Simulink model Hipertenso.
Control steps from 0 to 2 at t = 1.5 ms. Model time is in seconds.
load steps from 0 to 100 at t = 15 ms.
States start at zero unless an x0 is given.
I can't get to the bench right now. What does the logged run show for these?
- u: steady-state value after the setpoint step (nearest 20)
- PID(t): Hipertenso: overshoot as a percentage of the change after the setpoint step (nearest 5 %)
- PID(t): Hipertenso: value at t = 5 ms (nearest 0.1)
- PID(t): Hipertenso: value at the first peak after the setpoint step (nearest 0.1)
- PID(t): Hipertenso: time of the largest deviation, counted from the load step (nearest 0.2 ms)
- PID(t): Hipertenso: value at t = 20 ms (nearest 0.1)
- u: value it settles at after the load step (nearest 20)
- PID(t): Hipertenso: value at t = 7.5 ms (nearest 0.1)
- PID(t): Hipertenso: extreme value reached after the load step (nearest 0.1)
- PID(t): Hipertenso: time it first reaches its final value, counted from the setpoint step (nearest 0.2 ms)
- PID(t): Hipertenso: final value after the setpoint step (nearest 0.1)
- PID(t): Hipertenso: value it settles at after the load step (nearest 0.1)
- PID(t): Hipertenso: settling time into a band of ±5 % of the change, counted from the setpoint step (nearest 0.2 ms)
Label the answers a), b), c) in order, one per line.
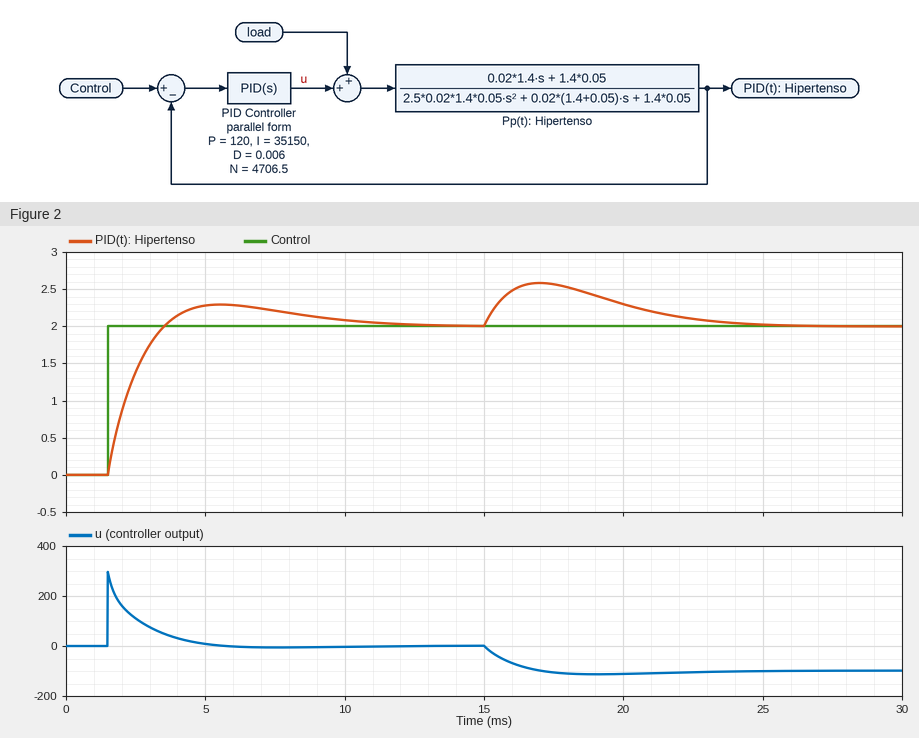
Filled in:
a) 0
b) 15 %
c) 2.3
d) 2.3
e) 2.0 ms
f) 2.3
g) -100
h) 2.2
i) 2.6
j) 2.0 ms
k) 2.0
l) 2.0
m) 8.0 ms
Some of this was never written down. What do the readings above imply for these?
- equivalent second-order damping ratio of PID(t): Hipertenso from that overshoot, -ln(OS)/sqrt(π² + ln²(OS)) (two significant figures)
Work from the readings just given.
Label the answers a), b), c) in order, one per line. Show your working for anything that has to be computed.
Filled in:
a) ln(0.15) = -1.897; 1.897 / sqrt(9.870 + 3.599) = 0.52
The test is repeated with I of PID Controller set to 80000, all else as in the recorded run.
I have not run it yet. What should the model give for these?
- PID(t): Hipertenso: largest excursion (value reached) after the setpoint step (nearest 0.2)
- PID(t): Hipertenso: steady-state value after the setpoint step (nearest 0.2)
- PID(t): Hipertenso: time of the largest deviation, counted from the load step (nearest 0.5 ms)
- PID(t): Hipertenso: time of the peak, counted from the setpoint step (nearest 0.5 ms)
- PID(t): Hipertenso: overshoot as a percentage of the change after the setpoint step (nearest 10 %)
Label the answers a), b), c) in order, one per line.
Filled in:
a) 2.4
b) 2.0
c) 1.5 ms
d) 3.0 ms
e) 20 %
